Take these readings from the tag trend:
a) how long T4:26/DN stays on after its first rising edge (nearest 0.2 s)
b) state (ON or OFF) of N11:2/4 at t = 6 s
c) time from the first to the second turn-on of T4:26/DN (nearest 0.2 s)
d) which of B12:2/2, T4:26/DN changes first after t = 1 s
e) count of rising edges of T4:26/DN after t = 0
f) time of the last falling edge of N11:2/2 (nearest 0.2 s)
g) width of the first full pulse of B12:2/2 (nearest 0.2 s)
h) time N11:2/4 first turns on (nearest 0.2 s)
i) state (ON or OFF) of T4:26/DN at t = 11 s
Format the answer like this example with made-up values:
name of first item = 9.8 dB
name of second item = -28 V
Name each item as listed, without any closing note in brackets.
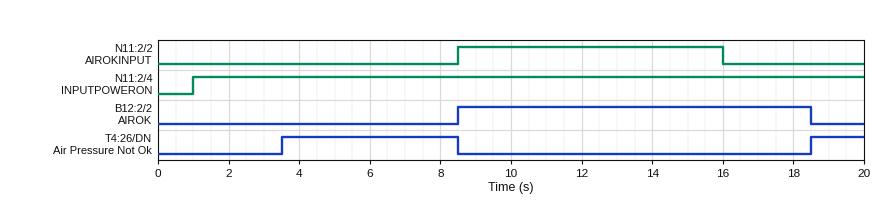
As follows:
how long T4:26/DN stays on after its first rising edge = 5.0 s
state (ON or OFF) of N11:2/4 at t = 6 s = ON
time from the first to the second turn-on of T4:26/DN = 15.0 s
which of B12:2/2, T4:26/DN changes first after t = 1 s = T4:26/DN
count of rising edges of T4:26/DN after t = 0 = 2
time of the last falling edge of N11:2/2 = 16.0 s
width of the first full pulse of B12:2/2 = 10.0 s
time N11:2/4 first turns on = 1.0 s
state (ON or OFF) of T4:26/DN at t = 11 s = OFF
